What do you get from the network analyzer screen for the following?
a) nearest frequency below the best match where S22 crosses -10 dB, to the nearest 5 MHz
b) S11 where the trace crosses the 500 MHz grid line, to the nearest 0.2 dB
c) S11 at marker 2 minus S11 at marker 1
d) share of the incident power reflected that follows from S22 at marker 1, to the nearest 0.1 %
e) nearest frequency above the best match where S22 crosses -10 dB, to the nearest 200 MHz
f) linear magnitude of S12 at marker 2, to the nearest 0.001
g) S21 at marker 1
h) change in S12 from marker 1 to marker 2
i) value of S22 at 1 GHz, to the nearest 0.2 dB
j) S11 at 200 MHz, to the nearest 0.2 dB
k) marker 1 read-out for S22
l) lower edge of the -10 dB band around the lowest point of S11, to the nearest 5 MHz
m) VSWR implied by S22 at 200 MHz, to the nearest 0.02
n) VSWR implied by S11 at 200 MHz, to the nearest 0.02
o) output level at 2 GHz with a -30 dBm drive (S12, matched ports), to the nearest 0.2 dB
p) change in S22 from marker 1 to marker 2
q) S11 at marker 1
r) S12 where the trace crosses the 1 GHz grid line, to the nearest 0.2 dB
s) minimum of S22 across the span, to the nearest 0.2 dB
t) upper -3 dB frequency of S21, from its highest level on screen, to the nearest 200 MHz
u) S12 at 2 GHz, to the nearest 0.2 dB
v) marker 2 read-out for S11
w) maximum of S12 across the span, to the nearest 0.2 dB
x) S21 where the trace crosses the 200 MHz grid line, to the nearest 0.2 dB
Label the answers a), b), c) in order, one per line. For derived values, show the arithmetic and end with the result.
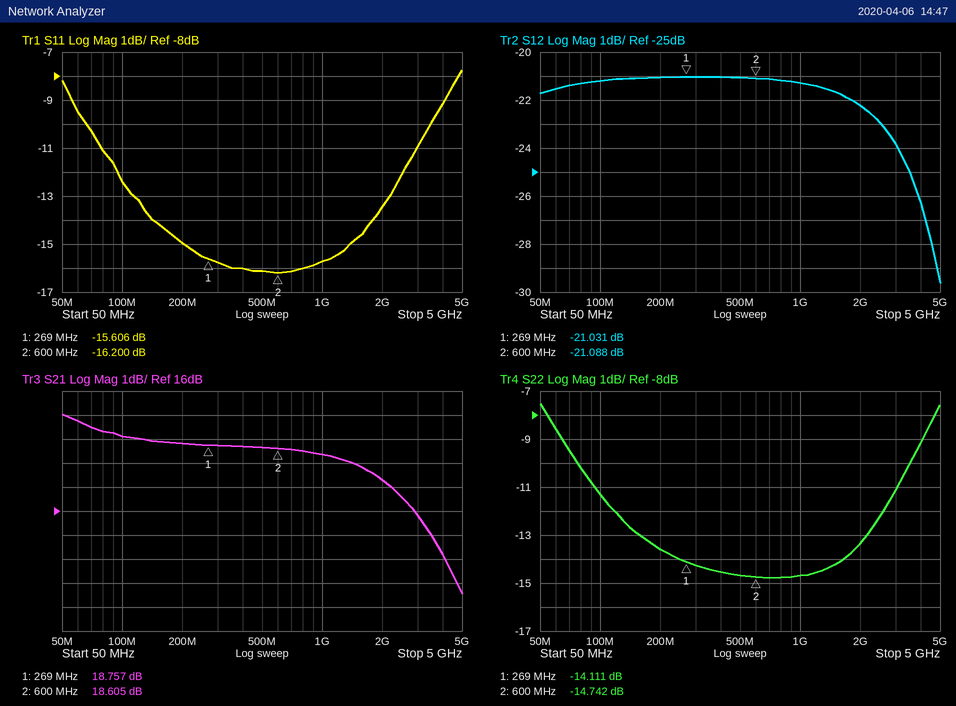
a) 75 MHz
b) -16.2 dB
c) -16.2 − (-15.606) = -0.594 dB
d) 10^(-14.111/10) ≈ 3.9 %
e) 3.6 GHz
f) 10^(-21.088/20) ≈ 0.088
g) 18.757 dB
h) -21.088 − (-21.031) = -0.057 dB
i) -14.6 dB
j) -15.0 dB
k) -14.111 dB
l) 65 MHz
m) |Γ| = 10^(-13.6/20) = 0.2089; VSWR = (1 + 0.2089)/(1 − 0.2089) ≈ 1.53, so 1.52 to the nearest 0.02
n) |Γ| = 10^(-15/20) = 0.1778; VSWR = (1 + 0.1778)/(1 − 0.1778) ≈ 1.43, so 1.44 to the nearest 0.02
o) -30 dBm + (-22.2 dB) = -52.2 dBm
p) -14.742 − (-14.111) = -0.631 dB
q) -15.606 dB
r) -21.2 dB
s) -14.8 dB
t) 2.2 GHz
u) -22.2 dB
v) -16.200 dB
w) -21.0 dB
x) 18.8 dB
